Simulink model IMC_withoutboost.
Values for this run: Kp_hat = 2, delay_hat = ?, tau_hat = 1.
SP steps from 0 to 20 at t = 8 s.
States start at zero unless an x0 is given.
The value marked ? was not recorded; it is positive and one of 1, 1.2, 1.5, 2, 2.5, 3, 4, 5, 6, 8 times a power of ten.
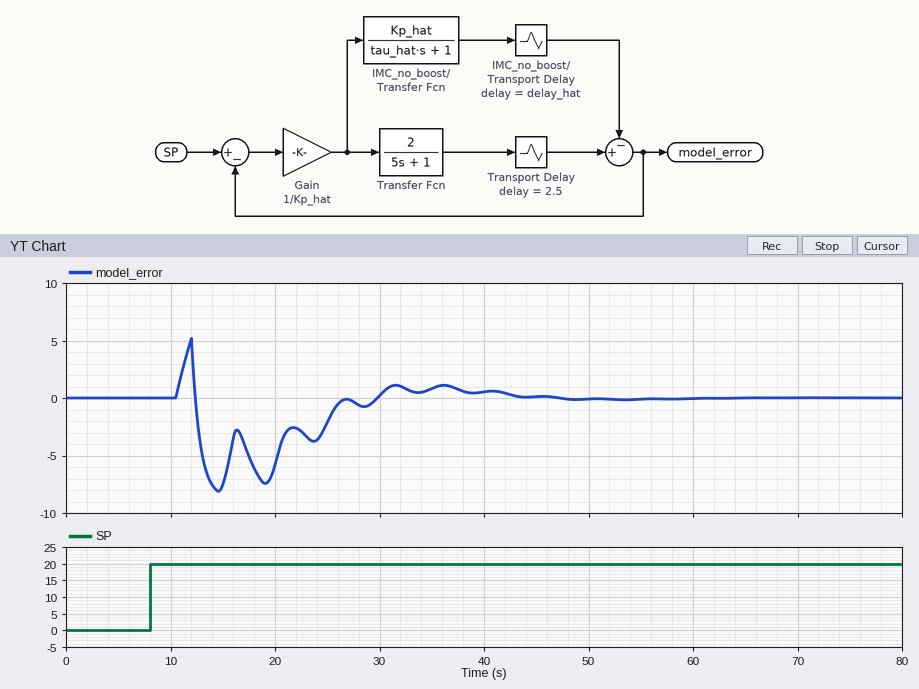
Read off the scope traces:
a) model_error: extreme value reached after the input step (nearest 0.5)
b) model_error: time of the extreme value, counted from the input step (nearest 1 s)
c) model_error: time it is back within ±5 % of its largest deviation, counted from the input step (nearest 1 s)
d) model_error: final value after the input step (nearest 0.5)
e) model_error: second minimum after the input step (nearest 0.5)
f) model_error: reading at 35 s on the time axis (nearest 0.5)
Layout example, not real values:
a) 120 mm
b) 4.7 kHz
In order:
a) -8.0
b) 7 s
c) 34 s
d) 0.0
e) -7.5
f) 1.0
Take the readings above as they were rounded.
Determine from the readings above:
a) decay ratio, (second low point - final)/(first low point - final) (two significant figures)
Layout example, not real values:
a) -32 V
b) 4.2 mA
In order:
a) 0.94
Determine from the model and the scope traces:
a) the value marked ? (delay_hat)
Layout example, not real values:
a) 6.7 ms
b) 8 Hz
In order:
a) 4
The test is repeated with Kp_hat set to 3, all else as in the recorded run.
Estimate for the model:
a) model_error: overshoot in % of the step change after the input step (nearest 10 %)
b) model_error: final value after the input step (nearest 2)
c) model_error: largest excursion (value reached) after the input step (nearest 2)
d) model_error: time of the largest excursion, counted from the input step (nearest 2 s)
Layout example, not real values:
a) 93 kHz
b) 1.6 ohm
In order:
a) 50 %
b) -10
c) -16
d) 12 s
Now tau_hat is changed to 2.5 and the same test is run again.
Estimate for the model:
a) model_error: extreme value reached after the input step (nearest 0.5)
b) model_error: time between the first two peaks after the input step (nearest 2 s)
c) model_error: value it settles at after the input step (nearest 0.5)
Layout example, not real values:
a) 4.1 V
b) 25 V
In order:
a) 5.0
b) 6 s
c) 0.0
